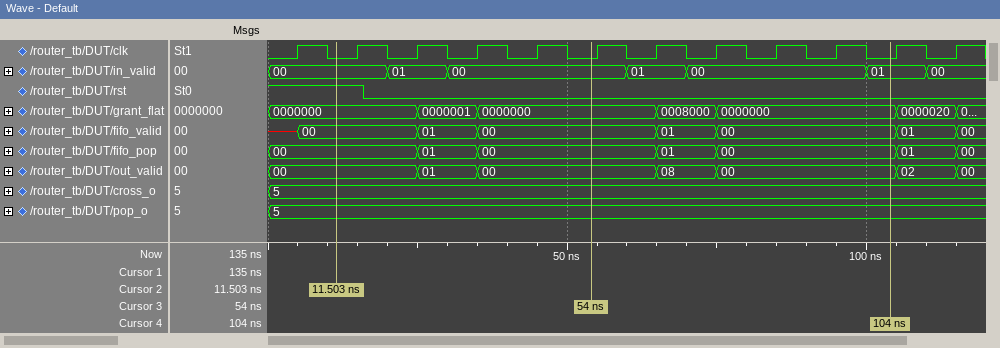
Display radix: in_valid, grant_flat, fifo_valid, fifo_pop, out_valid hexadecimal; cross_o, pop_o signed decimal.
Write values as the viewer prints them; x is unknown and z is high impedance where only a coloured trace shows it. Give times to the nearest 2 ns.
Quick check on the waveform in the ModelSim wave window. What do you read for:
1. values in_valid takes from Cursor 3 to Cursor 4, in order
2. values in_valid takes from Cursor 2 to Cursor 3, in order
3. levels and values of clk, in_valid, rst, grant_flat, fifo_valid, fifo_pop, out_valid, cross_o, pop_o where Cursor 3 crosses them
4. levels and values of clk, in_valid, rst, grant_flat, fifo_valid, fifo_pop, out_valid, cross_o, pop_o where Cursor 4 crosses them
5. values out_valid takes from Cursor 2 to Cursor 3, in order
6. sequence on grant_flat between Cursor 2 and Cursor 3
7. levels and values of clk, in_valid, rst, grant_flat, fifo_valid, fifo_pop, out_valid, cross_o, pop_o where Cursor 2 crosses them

00, 01, 00, 01
00, 01, 00
clk=0, in_valid=00, rst=0, grant_flat=0000000, fifo_valid=00, fifo_pop=00, out_valid=00, cross_o=5, pop_o=5
clk=0, in_valid=01, rst=0, grant_flat=0000000, fifo_valid=00, fifo_pop=00, out_valid=00, cross_o=5, pop_o=5
00, 01, 00
0000000, 0000001, 0000000
clk=0, in_valid=00, rst=1, grant_flat=0000000, fifo_valid=00, fifo_pop=00, out_valid=00, cross_o=5, pop_o=5
